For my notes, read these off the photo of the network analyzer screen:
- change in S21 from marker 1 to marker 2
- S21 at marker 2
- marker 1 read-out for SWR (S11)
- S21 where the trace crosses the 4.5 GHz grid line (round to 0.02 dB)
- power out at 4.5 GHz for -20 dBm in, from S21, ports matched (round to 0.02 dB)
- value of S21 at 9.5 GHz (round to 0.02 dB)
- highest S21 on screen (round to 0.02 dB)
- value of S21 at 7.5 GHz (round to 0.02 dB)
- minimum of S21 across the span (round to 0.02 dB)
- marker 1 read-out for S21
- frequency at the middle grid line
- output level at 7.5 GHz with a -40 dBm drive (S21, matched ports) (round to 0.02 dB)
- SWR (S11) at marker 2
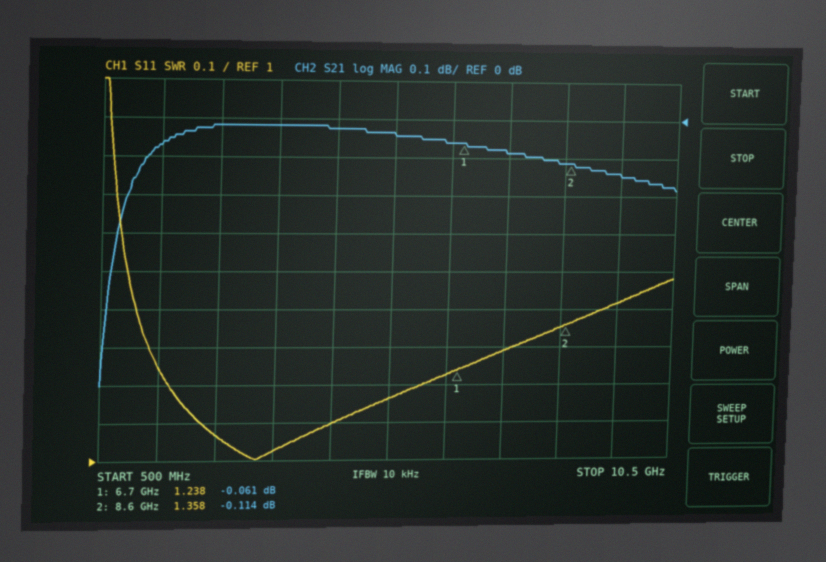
-0.053 dB
-0.114 dB
1.238
-0.02 dB
-20.02 dBm
-0.14 dB
-0.02 dB
-0.08 dB
-0.70 dB
-0.061 dB
5.5 GHz
-40.08 dBm
1.358
